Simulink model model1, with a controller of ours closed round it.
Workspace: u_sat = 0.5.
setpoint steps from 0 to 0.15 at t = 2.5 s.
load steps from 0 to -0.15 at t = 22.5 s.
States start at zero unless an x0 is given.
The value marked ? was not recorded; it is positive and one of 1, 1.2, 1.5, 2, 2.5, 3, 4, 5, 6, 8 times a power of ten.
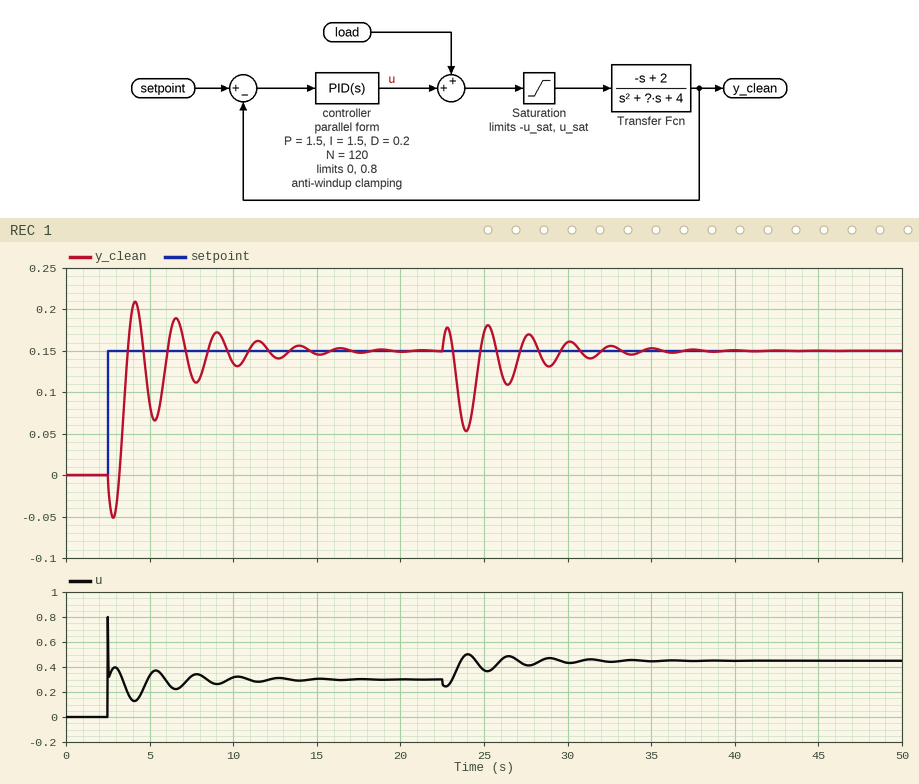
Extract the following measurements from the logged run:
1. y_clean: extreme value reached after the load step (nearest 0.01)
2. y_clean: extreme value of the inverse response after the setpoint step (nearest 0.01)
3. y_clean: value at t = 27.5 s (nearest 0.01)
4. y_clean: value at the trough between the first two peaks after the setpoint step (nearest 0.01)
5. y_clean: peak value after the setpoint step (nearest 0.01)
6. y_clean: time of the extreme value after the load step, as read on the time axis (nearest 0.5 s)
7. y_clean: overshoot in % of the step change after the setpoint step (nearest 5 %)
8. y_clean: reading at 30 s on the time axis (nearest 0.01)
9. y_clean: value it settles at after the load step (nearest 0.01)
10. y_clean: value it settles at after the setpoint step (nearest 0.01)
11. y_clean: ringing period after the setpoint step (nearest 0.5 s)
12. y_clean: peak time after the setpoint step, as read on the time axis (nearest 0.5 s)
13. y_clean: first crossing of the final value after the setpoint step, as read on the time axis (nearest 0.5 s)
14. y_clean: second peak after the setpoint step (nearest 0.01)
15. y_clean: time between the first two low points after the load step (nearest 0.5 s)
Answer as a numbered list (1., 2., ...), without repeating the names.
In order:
1. 0.05
2. -0.05
3. 0.17
4. 0.07
5. 0.21
6. 24.0 s
7. 40 %
8. 0.16
9. 0.15
10. 0.15
11. 2.5 s
12. 4.0 s
13. 3.5 s
14. 0.19
15. 2.5 s
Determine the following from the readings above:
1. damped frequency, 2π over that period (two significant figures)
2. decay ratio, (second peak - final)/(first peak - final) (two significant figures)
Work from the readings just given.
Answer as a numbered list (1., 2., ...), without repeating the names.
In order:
1. 2.5 rad/s
2. 0.67
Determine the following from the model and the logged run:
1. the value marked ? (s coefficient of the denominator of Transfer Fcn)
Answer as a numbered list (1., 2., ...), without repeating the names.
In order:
1. 2
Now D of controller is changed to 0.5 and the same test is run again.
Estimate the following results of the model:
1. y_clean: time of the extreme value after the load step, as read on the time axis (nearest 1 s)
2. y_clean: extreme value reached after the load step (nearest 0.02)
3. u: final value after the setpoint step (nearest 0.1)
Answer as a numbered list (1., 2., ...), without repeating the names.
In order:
1. 24 s
2. 0.08
3. 0.3
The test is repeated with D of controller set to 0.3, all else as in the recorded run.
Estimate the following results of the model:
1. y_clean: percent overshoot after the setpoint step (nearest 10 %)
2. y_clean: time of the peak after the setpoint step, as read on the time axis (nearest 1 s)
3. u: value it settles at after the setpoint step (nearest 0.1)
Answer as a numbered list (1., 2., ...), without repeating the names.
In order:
1. 30 %
2. 4 s
3. 0.3
